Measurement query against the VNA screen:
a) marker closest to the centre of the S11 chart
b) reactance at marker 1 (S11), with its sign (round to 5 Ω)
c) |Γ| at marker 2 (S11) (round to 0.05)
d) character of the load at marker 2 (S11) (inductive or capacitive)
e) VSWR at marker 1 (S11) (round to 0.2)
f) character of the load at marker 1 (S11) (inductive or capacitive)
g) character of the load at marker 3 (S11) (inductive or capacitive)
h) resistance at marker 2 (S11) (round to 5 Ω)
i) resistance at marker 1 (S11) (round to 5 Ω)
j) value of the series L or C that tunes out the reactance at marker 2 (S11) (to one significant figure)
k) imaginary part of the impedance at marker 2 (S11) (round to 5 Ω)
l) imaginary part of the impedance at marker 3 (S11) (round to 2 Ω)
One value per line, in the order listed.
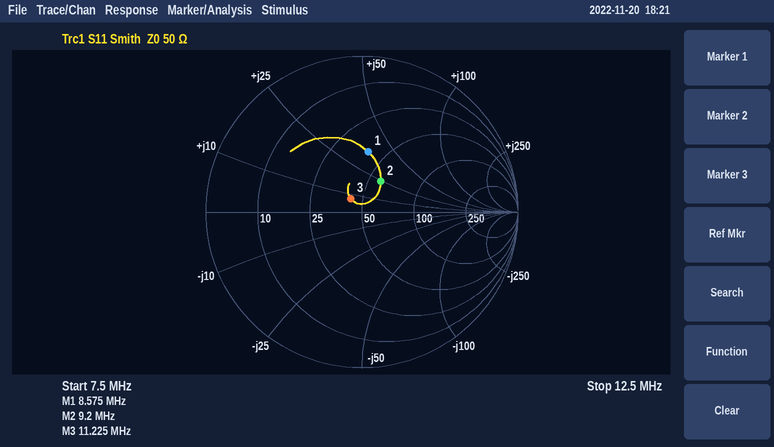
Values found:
marker 3
+35 Ω
0.25
inductive
2.2
inductive
inductive
60 Ω
40 Ω
700 pF
+25 Ω
+8 Ω
